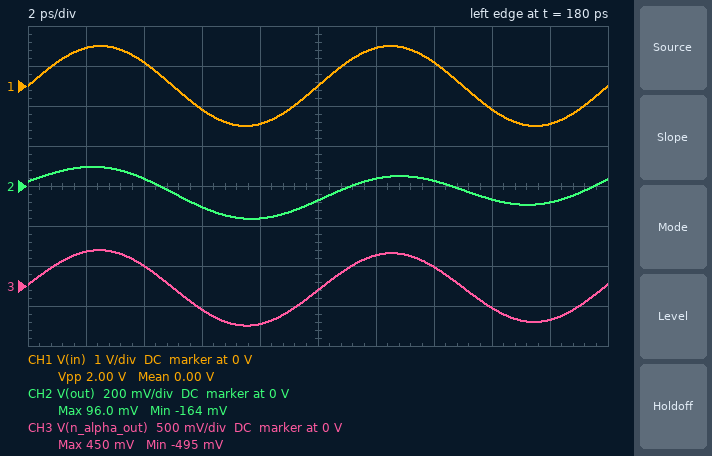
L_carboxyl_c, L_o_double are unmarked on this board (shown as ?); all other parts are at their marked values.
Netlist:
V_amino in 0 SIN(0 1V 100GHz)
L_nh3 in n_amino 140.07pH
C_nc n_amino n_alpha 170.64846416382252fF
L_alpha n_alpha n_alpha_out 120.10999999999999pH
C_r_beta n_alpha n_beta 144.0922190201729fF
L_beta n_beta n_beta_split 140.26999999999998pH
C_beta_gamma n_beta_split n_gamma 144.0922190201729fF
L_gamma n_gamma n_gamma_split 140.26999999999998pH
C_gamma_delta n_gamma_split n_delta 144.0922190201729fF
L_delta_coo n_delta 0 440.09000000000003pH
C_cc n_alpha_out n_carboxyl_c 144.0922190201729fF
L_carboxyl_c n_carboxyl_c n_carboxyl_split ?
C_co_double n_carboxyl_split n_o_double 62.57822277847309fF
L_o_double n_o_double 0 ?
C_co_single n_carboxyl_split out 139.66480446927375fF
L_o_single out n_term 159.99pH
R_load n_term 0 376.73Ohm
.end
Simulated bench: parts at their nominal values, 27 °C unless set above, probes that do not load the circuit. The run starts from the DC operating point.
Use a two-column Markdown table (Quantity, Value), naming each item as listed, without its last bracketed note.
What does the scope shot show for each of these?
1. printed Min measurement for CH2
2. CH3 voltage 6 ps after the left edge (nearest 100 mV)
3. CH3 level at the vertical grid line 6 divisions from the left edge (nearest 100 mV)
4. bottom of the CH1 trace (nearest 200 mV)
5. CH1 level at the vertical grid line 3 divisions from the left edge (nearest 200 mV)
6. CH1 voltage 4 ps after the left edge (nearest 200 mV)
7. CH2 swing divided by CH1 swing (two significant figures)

| Quantity | Value |
|---|---|
| printed Min measurement for CH2 | -164 mV |
| CH3 voltage 6 ps after the left edge | -300 mV |
| CH3 level at the vertical grid line 6 divisions from the left edge | 400 mV |
| bottom of the CH1 trace | -1.0 V |
| CH1 level at the vertical grid line 3 divisions from the left edge | -600 mV |
| CH1 voltage 4 ps after the left edge | 600 mV |
| CH2 swing divided by CH1 swing | 0.13 |
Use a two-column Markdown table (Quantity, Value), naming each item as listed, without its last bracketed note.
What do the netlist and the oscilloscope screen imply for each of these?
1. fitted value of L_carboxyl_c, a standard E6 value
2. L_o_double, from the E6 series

| Quantity | Value |
|---|---|
| fitted value of L_carboxyl_c, a standard E6 value | 220 pH |
| L_o_double, from the E6 series | 100 pH |
